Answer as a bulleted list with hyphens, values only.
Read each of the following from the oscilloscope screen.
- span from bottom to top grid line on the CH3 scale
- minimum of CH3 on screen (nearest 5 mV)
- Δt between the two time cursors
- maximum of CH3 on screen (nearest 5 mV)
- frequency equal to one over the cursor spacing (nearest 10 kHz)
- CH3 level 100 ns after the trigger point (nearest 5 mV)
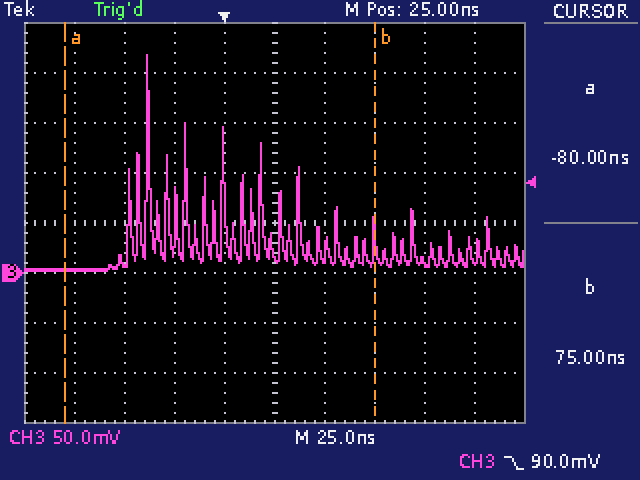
- 400 mV
- 0 mV
- 155.0 ns
- 220 mV
- 6.45 MHz
- 10 mV
